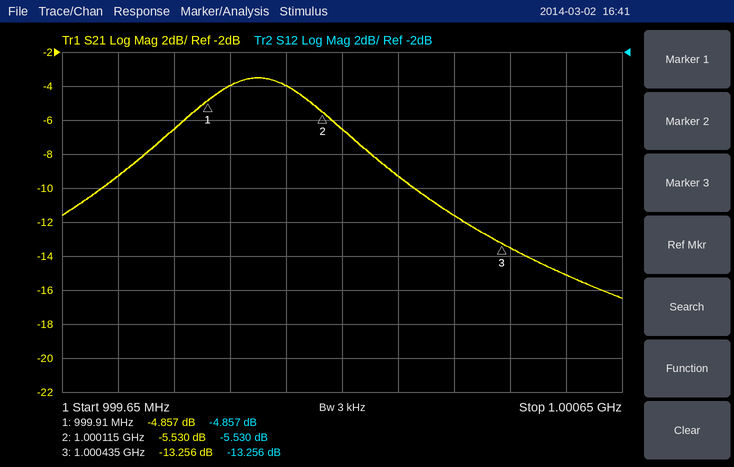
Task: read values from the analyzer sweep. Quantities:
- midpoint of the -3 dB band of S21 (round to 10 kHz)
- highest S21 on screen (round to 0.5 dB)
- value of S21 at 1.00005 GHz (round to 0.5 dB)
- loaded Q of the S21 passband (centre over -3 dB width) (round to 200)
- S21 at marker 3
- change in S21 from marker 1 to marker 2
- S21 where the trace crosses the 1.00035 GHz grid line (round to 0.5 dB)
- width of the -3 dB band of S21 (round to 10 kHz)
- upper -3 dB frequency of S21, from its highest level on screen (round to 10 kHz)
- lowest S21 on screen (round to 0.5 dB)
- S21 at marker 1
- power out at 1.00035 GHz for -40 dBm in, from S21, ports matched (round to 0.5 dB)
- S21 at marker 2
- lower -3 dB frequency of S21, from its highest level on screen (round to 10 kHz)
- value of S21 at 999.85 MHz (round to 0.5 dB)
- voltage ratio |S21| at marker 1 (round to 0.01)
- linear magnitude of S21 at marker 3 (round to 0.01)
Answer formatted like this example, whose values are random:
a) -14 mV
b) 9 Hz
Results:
a) 1.00000 GHz
b) -3.5 dB
c) -4.0 dB
d) 3400
e) -13.256 dB
f) -0.673 dB
g) -11.5 dB
h) 300 kHz
i) 1.00015 GHz
j) -16.5 dB
k) -4.857 dB
l) -51.5 dBm
m) -5.530 dB
n) 999.85 MHz
o) -6.5 dB
p) 0.57
q) 0.22
